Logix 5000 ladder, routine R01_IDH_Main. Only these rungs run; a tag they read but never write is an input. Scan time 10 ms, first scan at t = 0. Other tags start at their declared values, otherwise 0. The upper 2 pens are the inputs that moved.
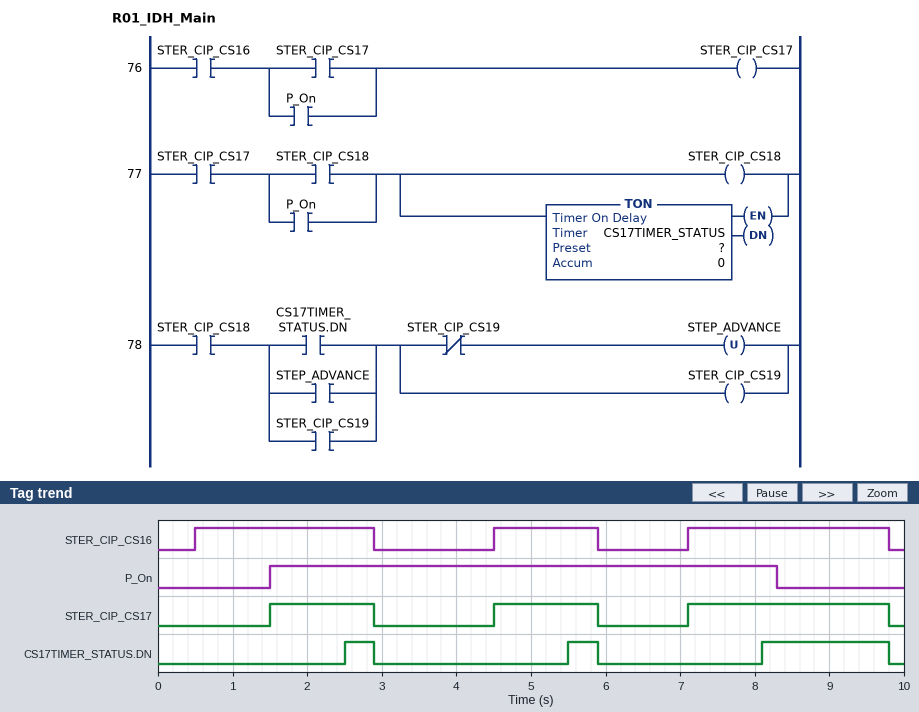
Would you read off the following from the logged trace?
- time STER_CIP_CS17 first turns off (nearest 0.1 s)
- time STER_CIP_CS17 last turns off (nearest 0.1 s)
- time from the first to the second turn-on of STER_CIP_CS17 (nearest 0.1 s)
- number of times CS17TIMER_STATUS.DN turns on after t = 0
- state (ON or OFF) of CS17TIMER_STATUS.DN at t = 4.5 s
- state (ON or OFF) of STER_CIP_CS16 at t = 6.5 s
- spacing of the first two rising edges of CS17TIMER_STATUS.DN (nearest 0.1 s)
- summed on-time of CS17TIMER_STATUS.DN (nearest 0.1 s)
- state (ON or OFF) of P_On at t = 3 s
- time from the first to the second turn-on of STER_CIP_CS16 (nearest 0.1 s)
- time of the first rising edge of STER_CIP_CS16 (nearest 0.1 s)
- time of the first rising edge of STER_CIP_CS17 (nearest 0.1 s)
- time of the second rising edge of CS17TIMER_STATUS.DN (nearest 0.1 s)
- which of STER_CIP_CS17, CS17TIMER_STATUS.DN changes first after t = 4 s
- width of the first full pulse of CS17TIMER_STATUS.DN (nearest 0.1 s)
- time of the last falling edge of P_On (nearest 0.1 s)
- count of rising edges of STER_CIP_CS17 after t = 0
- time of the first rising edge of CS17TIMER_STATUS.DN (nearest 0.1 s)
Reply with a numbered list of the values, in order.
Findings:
1. 2.9 s
2. 9.8 s
3. 3.0 s
4. 3
5. OFF
6. OFF
7. 3.0 s
8. 2.5 s
9. ON
10. 4.0 s
11. 0.5 s
12. 1.5 s
13. 5.5 s
14. STER_CIP_CS17
15. 0.4 s
16. 8.3 s
17. 3
18. 2.5 s
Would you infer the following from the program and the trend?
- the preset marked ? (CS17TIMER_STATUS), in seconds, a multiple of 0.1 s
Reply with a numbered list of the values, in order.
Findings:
1. 1.0 s
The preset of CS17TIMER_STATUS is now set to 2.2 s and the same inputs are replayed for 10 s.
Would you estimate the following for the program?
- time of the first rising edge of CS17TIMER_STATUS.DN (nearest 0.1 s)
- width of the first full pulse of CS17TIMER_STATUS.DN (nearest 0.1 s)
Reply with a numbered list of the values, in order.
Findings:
1. 9.3 s
2. 0.5 s
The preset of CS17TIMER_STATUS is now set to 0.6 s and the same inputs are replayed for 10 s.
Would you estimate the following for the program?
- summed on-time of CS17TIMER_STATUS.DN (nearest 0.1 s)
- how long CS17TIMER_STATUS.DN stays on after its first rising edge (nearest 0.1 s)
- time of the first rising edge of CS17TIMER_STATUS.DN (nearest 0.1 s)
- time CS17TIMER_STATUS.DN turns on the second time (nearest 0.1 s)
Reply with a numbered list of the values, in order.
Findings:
1. 3.7 s
2. 0.8 s
3. 2.1 s
4. 5.1 s
